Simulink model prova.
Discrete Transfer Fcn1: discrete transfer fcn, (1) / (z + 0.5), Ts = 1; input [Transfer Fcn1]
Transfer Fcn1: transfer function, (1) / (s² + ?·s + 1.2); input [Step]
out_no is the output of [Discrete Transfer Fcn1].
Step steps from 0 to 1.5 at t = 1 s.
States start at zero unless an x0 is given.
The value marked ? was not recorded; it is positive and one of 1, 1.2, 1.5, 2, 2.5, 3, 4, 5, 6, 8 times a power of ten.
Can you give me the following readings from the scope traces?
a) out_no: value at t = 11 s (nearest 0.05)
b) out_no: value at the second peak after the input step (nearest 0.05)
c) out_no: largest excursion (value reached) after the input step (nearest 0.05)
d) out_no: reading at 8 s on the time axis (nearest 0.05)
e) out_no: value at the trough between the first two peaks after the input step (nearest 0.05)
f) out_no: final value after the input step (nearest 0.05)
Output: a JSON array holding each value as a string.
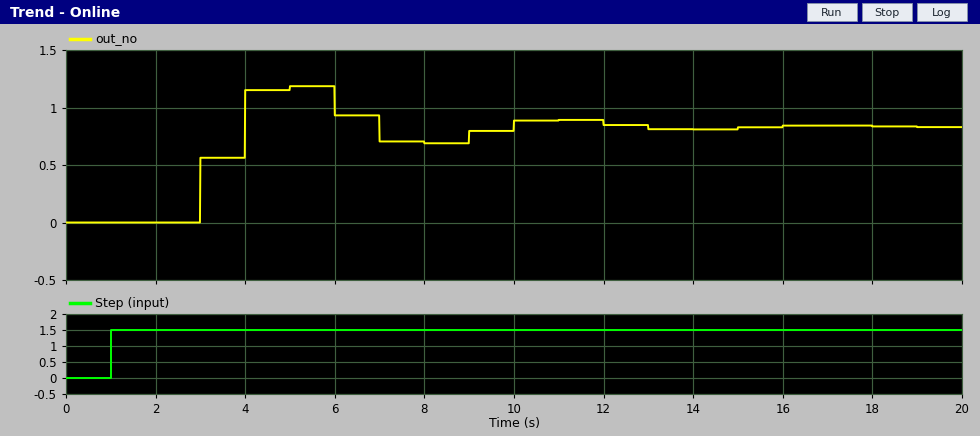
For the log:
["0.90", "0.90", "1.20", "0.70", "0.70", "0.85"]
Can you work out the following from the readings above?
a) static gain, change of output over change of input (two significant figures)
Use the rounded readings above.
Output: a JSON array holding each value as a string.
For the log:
["0.57"]
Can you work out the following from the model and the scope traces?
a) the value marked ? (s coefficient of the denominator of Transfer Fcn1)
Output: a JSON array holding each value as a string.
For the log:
["0.6"]
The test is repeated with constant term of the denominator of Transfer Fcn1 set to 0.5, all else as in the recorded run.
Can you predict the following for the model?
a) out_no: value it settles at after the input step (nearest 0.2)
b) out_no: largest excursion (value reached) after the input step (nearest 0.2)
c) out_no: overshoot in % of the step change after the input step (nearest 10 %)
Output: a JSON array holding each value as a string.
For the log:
["2.0", "2.4", "20 %"]
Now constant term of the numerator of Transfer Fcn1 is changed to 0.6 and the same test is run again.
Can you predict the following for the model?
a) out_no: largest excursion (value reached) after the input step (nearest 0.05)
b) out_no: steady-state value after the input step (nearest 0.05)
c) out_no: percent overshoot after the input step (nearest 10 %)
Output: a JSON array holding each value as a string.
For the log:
["0.70", "0.50", "40 %"]
